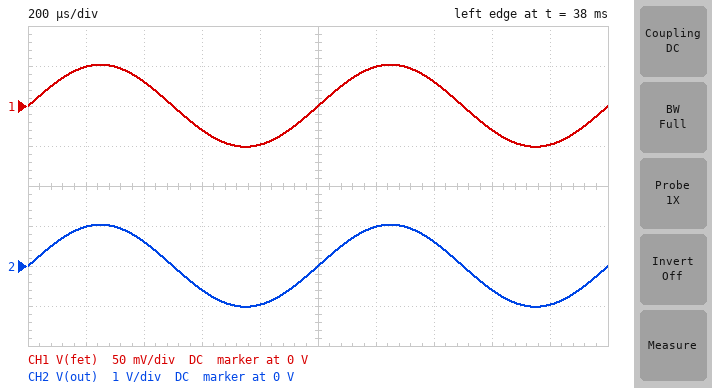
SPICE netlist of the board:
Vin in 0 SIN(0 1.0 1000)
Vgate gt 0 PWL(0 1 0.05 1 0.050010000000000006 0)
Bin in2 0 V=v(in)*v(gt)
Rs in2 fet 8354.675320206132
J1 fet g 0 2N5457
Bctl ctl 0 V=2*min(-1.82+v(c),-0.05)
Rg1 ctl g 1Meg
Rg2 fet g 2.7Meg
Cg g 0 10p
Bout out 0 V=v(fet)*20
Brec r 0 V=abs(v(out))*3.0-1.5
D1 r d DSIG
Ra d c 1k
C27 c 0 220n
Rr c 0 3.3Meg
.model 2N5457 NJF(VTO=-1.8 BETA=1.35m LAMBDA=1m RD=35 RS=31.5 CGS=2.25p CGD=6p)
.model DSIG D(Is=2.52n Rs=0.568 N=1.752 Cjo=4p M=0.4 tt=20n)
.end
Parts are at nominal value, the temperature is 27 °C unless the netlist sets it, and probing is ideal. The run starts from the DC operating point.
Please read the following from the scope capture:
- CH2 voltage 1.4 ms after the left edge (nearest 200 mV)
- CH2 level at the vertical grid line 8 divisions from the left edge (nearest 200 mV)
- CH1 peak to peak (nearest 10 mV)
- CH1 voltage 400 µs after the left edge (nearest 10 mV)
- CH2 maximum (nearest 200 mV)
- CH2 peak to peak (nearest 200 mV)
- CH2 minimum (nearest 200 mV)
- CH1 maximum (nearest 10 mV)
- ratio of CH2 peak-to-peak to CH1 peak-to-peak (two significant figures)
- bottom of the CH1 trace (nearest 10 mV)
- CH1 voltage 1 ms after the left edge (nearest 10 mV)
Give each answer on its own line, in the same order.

600 mV
-600 mV
100 mV
30 mV
1.0 V
2.0 V
-1.0 V
50 mV
20
-50 mV
0 V
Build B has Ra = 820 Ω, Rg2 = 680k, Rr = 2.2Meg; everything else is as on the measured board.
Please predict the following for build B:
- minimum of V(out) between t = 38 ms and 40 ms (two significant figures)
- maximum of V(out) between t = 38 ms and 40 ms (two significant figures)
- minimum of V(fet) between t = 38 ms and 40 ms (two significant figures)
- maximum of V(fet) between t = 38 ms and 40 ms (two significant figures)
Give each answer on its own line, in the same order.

-940 mV
910 mV
-47 mV
46 mV
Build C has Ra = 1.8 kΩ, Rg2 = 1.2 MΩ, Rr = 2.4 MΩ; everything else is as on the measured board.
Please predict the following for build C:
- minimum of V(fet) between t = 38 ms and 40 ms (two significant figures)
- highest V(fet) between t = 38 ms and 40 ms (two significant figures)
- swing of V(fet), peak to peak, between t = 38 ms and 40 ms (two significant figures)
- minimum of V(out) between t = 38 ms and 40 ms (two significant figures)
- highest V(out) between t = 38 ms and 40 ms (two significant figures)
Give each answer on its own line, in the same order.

-49 mV
49 mV
98 mV
-990 mV
980 mV
